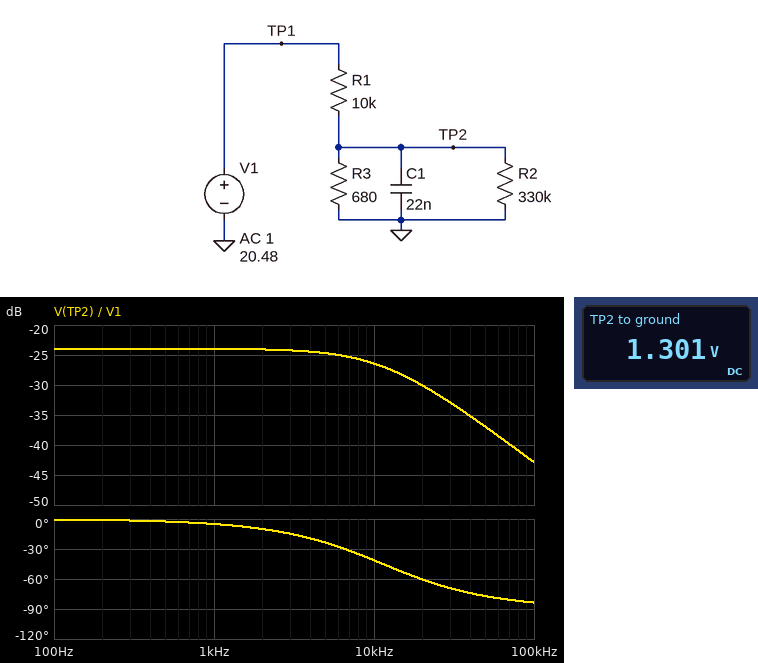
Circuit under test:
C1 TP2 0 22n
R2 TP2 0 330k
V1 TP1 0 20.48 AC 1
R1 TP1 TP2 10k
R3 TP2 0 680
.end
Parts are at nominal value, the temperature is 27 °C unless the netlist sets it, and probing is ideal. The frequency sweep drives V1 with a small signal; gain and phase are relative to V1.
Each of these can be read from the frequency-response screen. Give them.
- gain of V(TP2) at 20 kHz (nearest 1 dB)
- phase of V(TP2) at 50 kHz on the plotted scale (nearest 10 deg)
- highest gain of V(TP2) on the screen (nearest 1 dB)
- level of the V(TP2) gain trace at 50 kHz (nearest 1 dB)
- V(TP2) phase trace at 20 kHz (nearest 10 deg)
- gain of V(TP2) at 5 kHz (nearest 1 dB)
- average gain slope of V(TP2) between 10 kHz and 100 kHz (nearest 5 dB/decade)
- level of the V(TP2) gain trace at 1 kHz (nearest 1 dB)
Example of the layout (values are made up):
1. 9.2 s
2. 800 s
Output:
1. -30 dB
2. -80 deg
3. -24 dB
4. -37 dB
5. -60 deg
6. -25 dB
7. -15 dB/decade
8. -24 dB
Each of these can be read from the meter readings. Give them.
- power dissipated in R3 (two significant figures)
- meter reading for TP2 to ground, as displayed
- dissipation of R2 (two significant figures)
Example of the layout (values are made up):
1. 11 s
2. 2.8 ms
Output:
1. 2.5 mW
2. 1.301 V
3. 5.1 µW
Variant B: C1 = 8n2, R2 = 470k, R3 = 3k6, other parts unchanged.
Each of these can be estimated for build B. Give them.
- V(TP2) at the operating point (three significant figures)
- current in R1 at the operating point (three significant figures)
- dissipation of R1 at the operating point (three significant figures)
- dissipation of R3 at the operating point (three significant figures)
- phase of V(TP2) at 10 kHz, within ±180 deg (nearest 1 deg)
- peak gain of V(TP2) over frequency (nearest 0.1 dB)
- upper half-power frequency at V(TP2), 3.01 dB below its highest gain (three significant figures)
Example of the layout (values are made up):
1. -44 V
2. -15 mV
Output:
1. 5.39 V
2. 1.51 mA
3. 22.8 mW
4. 8.07 mW
5. -54 deg
6. -11.6 dB
7. 7.37 kHz
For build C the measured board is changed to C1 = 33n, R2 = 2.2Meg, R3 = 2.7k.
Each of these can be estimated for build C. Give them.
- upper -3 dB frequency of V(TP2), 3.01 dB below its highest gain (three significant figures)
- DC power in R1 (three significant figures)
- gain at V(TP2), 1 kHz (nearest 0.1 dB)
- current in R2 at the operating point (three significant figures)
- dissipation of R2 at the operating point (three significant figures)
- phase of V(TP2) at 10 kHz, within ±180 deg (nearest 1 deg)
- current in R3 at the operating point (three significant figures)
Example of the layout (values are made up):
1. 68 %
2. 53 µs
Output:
1. 2.27 kHz
2. 26.0 mW
3. -14.2 dB
4. 1.98 µA
5. 8.60 µW
6. -77 deg
7. 1.61 mA
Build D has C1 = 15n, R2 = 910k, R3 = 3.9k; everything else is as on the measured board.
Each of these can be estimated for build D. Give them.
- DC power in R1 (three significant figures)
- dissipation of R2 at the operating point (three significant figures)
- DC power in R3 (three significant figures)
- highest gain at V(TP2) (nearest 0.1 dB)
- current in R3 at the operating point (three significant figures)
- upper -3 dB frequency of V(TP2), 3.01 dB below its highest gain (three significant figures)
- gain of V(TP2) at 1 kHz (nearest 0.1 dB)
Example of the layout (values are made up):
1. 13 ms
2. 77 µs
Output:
1. 21.8 mW
2. 36.1 µW
3. 8.41 mW
4. -11.1 dB
5. 1.47 mA
6. 3.79 kHz
7. -11.4 dB
